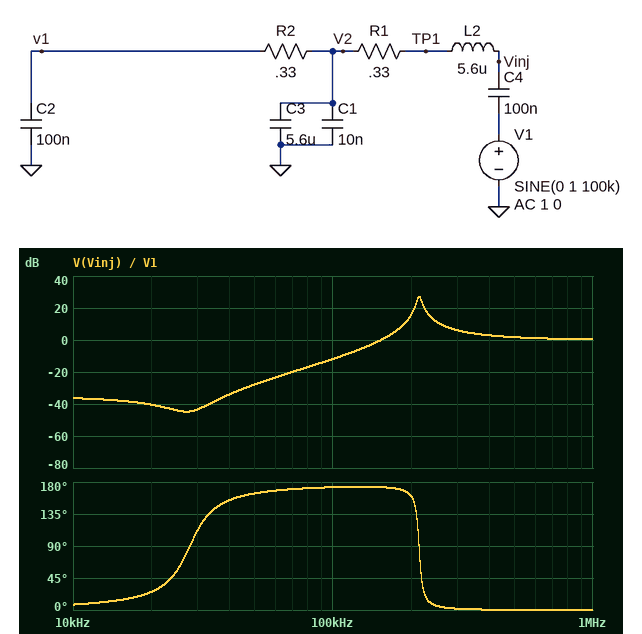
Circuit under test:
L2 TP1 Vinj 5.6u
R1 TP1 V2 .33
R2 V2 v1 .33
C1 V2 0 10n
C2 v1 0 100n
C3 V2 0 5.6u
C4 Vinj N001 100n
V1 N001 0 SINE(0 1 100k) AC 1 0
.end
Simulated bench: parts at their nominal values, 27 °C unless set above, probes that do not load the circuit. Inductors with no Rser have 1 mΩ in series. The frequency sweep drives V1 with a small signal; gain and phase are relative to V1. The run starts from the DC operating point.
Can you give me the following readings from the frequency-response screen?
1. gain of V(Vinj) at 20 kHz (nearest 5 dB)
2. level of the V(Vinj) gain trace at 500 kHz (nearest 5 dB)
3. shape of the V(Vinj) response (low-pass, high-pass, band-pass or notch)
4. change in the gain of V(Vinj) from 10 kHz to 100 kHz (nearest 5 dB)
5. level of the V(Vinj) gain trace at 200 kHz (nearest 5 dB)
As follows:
-40 dB
0 dB
band-pass
25 dB
15 dB
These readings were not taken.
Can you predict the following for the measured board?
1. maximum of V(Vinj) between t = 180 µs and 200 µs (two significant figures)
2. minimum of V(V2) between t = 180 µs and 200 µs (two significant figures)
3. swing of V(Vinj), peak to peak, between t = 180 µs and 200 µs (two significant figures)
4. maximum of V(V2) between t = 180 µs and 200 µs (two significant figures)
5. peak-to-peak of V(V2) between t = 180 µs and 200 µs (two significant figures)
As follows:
260 mV
-22 mV
510 mV
22 mV
44 mV
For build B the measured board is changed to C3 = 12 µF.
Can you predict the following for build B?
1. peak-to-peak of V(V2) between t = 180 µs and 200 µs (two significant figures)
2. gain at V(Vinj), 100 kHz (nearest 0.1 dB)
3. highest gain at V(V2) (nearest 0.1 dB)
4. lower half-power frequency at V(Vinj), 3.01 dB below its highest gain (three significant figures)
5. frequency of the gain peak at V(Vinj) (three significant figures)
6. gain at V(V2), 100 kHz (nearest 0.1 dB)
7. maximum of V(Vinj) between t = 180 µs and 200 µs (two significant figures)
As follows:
21 mV
-11.3 dB
-14.6 dB
209 kHz
214 kHz
-39.6 dB
270 mV
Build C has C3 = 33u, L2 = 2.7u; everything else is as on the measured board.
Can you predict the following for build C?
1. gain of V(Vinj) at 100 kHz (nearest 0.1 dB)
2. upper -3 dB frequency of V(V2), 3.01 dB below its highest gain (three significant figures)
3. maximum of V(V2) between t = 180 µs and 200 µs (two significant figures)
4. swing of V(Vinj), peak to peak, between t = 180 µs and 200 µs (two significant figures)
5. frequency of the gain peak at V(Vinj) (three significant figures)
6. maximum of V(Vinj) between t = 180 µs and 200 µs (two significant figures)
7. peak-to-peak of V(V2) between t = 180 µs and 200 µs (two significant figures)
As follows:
-18.6 dB
316 kHz
3.4 mV
240 mV
307 kHz
120 mV
6.7 mV
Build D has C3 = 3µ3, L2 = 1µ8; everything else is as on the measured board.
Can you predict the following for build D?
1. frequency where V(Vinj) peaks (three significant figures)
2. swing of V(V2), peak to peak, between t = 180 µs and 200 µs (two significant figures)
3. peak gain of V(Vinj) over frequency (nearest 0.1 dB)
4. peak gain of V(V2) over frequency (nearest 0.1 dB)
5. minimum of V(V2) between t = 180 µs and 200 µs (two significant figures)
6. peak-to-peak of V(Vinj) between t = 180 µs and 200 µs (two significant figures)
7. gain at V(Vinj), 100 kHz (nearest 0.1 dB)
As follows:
381 kHz
61 mV
22.1 dB
-8.6 dB
-31 mV
97 mV
-26.3 dB
